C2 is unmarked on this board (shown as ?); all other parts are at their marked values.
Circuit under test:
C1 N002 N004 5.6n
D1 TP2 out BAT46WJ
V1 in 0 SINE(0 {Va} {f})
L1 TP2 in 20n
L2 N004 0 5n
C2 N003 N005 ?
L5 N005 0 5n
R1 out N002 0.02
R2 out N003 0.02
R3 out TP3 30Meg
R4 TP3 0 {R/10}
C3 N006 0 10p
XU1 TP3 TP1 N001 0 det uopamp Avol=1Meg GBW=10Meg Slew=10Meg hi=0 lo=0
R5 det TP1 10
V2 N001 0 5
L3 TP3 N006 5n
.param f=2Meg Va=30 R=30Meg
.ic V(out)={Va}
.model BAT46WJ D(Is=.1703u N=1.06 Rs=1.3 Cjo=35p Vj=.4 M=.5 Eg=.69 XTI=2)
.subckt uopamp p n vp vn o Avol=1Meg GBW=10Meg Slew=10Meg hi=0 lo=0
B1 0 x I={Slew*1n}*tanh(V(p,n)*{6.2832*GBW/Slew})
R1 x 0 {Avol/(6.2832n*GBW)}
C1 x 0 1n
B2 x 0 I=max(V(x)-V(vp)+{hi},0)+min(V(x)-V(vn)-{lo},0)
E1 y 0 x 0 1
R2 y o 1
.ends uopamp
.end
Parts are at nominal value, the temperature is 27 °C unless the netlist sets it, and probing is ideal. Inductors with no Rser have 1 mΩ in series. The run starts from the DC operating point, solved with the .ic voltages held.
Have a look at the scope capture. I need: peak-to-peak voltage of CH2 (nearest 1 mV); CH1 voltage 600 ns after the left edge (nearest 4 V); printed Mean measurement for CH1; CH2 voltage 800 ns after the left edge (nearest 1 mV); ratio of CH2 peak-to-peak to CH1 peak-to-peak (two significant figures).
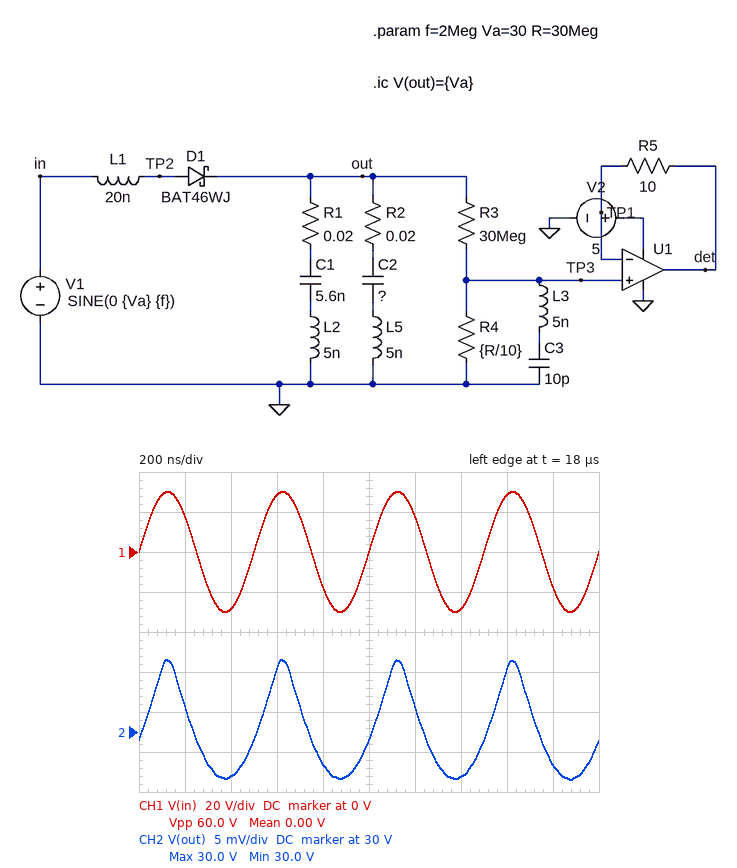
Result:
15 mV
28 V
0.00 V
29.996 V
0.00025
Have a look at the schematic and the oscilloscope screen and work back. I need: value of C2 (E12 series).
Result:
15 nF
